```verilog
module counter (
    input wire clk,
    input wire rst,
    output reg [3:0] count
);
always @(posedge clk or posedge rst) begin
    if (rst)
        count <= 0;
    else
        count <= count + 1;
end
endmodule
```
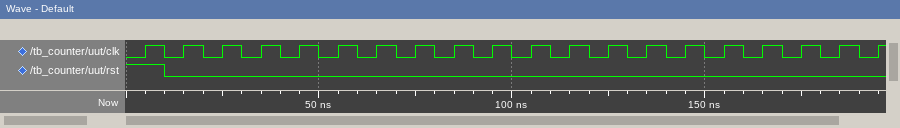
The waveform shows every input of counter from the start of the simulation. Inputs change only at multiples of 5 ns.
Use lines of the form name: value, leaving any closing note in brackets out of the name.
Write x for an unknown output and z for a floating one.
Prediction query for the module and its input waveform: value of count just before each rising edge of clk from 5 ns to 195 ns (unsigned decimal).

value of count just before each rising edge of clk from 5 ns to 195 ns: 0, 0, 1, 2, 3, 4, 5, 6, 7, 8, 9, 10, 11, 12, 13, 14, 15, 0, 1, 2
